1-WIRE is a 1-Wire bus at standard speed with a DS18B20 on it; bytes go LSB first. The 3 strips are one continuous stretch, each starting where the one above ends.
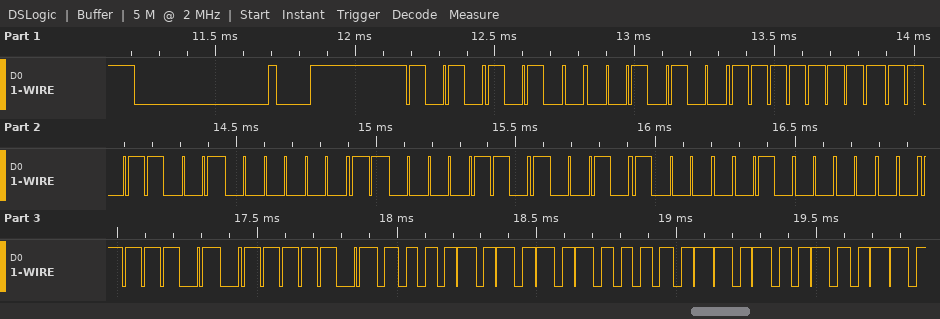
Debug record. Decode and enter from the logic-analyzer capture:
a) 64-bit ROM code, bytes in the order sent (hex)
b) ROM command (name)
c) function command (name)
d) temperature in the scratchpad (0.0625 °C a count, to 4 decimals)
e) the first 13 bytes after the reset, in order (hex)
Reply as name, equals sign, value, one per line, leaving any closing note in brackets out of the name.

64-bit ROM code, bytes in the order sent = 28 FF 9B C0 B0 14 04 BC
ROM command = Match ROM
function command = Read Scratchpad
temperature in the scratchpad = 85.0000 °C
the first 13 bytes after the reset, in order = 55 28 FF 9B C0 B0 14 04 BC BE 50 05 4B
